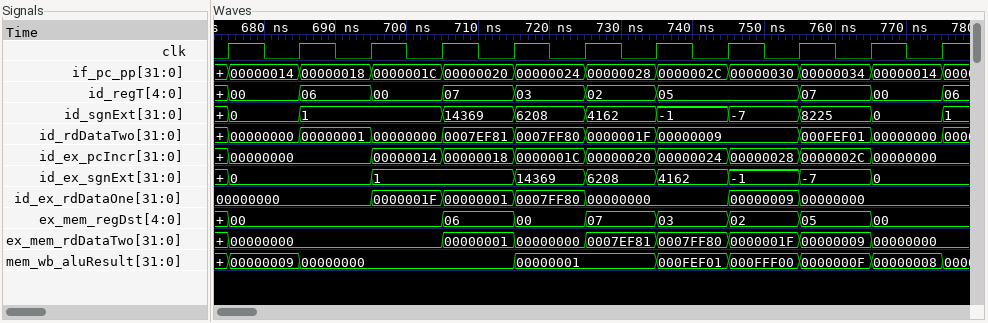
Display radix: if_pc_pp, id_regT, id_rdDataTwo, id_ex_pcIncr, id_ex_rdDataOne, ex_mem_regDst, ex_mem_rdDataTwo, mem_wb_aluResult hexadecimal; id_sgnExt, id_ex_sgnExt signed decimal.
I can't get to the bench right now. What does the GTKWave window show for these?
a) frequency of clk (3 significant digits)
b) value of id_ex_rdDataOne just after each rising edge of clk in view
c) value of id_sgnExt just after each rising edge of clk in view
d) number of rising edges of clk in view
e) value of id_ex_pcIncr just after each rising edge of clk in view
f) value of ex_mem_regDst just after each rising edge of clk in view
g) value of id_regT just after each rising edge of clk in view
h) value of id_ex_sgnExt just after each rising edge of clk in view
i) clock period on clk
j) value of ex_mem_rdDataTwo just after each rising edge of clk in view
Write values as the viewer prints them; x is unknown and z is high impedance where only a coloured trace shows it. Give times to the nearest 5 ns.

100 MHz
00000000, 00000000, 0000001F, 00000001, 0007FF80, 00000000, 00000000, 00000009, 00000000, 00000000, 00000000
0, 1, 1, 14369, 6208, 4162, -1, -7, 8225, 0, 1
11
00000000, 00000000, 00000014, 00000018, 0000001C, 00000020, 00000024, 00000028, 0000002C, 00000000, 00000000
00, 00, 00, 06, 00, 07, 03, 02, 05, 00, 00
00, 06, 00, 07, 03, 02, 05, 05, 07, 00, 06
0, 0, 1, 1, 14369, 6208, 4162, -1, -7, 0, 0
10 ns
00000000, 00000000, 00000000, 00000001, 00000000, 0007EF81, 0007FF80, 0000001F, 00000009, 00000000, 00000000
